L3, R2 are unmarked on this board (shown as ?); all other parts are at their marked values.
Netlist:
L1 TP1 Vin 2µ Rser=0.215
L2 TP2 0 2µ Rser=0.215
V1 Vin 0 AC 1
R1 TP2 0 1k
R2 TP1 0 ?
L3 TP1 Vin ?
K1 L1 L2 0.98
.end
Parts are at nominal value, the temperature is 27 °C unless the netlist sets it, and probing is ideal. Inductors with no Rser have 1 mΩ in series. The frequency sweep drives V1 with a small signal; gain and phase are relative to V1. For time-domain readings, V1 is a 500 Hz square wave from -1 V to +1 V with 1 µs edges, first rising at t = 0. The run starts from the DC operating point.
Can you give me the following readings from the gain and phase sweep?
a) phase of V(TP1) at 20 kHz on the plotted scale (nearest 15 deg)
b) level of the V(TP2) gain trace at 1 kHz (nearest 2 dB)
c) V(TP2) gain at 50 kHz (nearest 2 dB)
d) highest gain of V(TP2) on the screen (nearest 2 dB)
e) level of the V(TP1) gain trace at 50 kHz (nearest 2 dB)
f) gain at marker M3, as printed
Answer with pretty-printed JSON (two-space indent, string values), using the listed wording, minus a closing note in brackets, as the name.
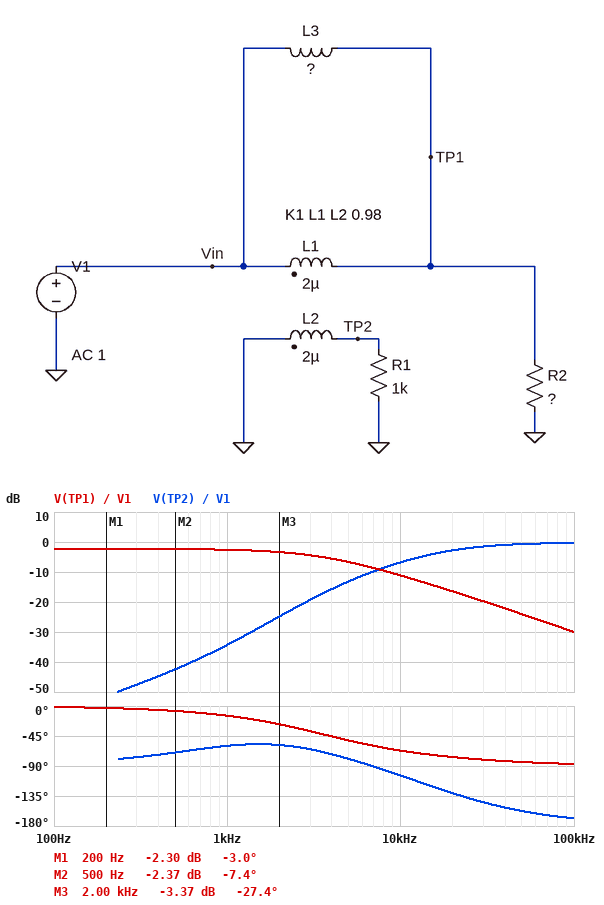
{
  "phase of V(TP1) at 20 kHz on the plotted scale": "-75 deg",
  "level of the V(TP2) gain trace at 1 kHz": "-34 dB",
  "V(TP2) gain at 50 kHz": "0 dB",
  "highest gain of V(TP2) on the screen": "0 dB",
  "level of the V(TP1) gain trace at 50 kHz": "-24 dB",
  "gain at marker M3, as printed": "-3.37 dB"
}
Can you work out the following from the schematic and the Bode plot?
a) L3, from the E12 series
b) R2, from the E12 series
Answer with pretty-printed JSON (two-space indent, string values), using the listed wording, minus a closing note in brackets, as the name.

{
  "L3, from the E12 series": "180 nH",
  "R2, from the E12 series": "3.3 mΩ"
}
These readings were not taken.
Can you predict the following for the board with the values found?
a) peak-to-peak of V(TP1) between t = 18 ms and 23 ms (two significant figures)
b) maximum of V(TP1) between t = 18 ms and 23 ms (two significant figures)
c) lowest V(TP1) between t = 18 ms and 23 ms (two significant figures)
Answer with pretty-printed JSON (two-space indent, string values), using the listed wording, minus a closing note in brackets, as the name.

{
  "peak-to-peak of V(TP1) between t = 18 ms and 23 ms": "1.5 V",
  "maximum of V(TP1) between t = 18 ms and 23 ms": "770 mV",
  "lowest V(TP1) between t = 18 ms and 23 ms": "-770 mV"
}
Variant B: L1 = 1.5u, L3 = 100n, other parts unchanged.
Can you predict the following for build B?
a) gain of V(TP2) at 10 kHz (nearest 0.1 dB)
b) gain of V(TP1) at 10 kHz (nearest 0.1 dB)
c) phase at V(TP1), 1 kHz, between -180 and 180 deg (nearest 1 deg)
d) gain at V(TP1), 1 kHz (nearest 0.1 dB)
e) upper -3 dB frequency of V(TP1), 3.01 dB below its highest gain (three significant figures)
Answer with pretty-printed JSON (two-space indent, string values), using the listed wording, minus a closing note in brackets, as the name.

{
  "gain of V(TP2) at 10 kHz": "-8.5 dB",
  "gain of V(TP1) at 10 kHz": "-7.2 dB",
  "phase at V(TP1), 1 kHz, between -180 and 180 deg": "-8 deg",
  "gain at V(TP1), 1 kHz": "-2.4 dB",
  "upper -3 dB frequency of V(TP1), 3.01 dB below its highest gain": "6.82 kHz"
}
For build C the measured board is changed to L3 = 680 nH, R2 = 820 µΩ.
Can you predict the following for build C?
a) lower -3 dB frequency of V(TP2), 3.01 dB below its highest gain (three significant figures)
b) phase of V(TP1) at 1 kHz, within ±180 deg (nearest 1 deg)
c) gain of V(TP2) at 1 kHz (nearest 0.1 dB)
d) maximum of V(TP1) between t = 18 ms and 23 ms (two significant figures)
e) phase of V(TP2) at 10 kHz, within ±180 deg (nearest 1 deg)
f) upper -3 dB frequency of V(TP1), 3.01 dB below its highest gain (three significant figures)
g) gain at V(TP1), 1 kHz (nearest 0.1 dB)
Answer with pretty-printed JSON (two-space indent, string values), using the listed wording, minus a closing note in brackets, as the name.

{
  "lower -3 dB frequency of V(TP2), 3.01 dB below its highest gain": "17.2 kHz",
  "phase of V(TP1) at 1 kHz, within ±180 deg": "-66 deg",
  "gain of V(TP2) at 1 kHz": "-25.4 dB",
  "maximum of V(TP1) between t = 18 ms and 23 ms": "390 mV",
  "phase of V(TP2) at 10 kHz, within ±180 deg": "-119 deg",
  "upper -3 dB frequency of V(TP1), 3.01 dB below its highest gain": "425 Hz",
  "gain at V(TP1), 1 kHz": "-15.0 dB"
}
